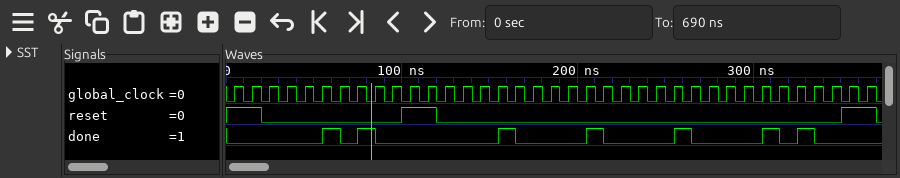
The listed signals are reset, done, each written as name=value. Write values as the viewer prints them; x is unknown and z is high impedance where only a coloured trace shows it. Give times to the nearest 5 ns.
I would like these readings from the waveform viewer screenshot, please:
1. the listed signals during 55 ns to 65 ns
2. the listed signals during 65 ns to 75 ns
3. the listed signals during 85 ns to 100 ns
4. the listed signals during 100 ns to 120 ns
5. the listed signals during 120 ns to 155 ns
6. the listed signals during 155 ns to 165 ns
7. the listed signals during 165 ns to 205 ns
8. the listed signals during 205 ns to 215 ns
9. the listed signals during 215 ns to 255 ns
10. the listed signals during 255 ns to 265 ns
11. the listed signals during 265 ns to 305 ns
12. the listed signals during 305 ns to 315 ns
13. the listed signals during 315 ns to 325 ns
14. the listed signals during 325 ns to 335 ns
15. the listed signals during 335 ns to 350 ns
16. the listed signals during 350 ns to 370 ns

reset=0, done=1
reset=0, done=0
reset=0, done=0
reset=1, done=0
reset=0, done=0
reset=0, done=1
reset=0, done=0
reset=0, done=1
reset=0, done=0
reset=0, done=1
reset=0, done=0
reset=0, done=1
reset=0, done=0
reset=0, done=1
reset=0, done=0
reset=1, done=0
